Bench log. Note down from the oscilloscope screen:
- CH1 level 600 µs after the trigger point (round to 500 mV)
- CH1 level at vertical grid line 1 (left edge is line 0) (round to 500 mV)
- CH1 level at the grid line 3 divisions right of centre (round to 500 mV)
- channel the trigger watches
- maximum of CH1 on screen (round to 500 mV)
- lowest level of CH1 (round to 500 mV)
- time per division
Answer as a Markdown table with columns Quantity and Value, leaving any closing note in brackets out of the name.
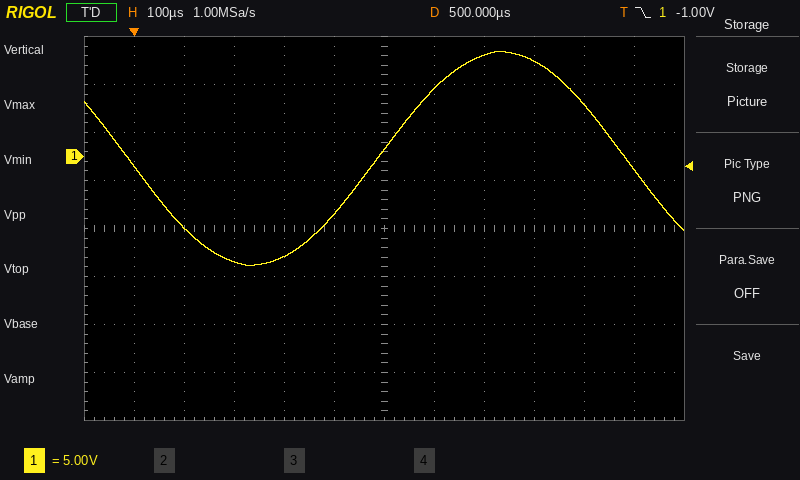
| Quantity | Value |
|---|---|
| CH1 level 600 µs after the trigger point | 7.0 V |
| CH1 level at vertical grid line 1 (left edge is line 0) | -1.0 V |
| CH1 level at the grid line 3 divisions right of centre | 10.0 V |
| channel the trigger watches | CH1 |
| maximum of CH1 on screen | 11.0 V |
| lowest level of CH1 | -11.5 V |
| time per division | 100 µs |
